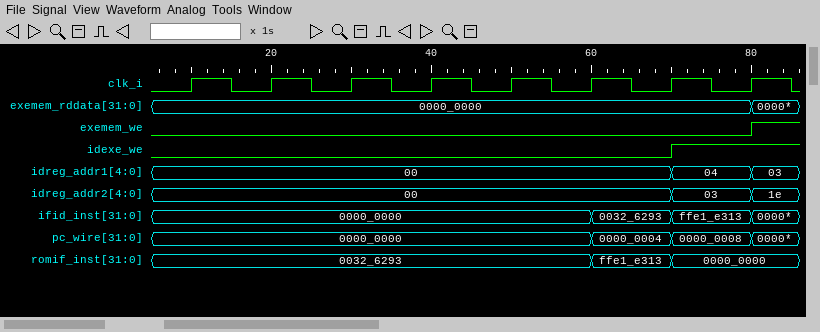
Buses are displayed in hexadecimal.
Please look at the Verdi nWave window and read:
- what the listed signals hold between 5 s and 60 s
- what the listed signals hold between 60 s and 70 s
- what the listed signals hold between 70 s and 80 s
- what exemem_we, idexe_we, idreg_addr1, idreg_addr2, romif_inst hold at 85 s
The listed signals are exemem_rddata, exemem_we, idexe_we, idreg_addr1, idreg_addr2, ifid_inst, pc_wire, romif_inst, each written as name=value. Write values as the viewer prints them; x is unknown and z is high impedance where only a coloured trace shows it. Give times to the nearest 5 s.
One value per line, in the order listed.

exemem_rddata=0000_0000, exemem_we=0, idexe_we=0, idreg_addr1=00, idreg_addr2=00, ifid_inst=0000_0000, pc_wire=0000_0000, romif_inst=0032_6293
exemem_rddata=0000_0000, exemem_we=0, idexe_we=0, idreg_addr1=00, idreg_addr2=00, ifid_inst=0032_6293, pc_wire=0000_0004, romif_inst=ffe1_e313
exemem_rddata=0000_0000, exemem_we=0, idexe_we=1, idreg_addr1=04, idreg_addr2=03, ifid_inst=ffe1_e313, pc_wire=0000_0008, romif_inst=0000_0000
exemem_we=1, idexe_we=1, idreg_addr1=03, idreg_addr2=1e, romif_inst=0000_0000
